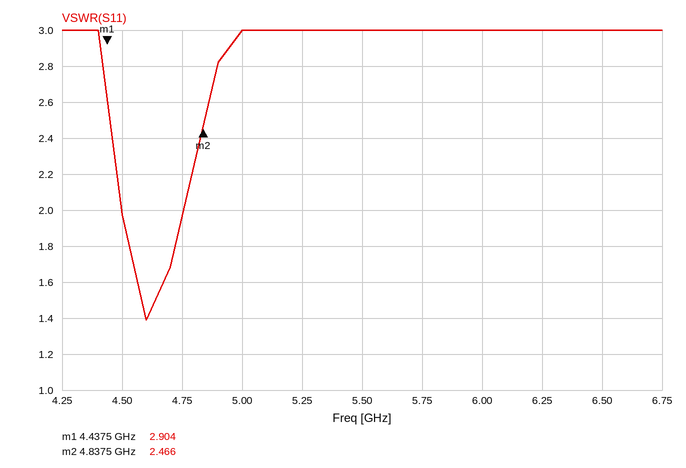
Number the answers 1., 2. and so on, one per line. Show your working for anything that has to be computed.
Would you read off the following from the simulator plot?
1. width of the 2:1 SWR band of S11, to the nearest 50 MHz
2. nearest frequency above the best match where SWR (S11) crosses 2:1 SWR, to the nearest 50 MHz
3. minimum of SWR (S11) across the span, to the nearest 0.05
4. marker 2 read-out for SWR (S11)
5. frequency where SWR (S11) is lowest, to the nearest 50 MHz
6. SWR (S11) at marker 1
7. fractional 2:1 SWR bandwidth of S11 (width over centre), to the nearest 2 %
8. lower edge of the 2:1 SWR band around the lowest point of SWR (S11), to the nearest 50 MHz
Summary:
1. 4.75 GHz − 4.50 GHz = 250 MHz
2. 4.75 GHz
3. 1.40
4. 2.466
5. 4.60 GHz
6. 2.904
7. 250 MHz / 4.625 GHz ≈ 5.41 %, so 6 % to the nearest 2 %
8. 4.50 GHz
